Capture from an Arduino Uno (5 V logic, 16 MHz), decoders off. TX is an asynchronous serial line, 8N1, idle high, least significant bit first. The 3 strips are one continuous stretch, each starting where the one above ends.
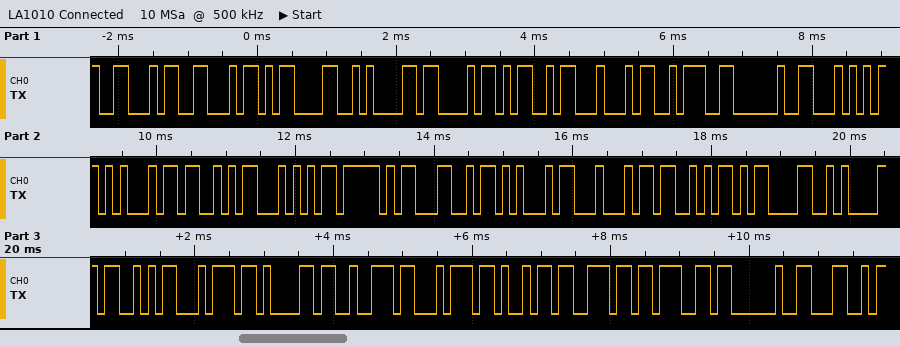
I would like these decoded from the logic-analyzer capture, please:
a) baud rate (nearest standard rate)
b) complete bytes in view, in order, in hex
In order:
9600 baud
46 46 0D 0A 43 4D 44 3A 20 54 45 53 54 5F 4C 45 44 53 0D 0A 53 74 61 72 74 69 6E 67 20 4C
